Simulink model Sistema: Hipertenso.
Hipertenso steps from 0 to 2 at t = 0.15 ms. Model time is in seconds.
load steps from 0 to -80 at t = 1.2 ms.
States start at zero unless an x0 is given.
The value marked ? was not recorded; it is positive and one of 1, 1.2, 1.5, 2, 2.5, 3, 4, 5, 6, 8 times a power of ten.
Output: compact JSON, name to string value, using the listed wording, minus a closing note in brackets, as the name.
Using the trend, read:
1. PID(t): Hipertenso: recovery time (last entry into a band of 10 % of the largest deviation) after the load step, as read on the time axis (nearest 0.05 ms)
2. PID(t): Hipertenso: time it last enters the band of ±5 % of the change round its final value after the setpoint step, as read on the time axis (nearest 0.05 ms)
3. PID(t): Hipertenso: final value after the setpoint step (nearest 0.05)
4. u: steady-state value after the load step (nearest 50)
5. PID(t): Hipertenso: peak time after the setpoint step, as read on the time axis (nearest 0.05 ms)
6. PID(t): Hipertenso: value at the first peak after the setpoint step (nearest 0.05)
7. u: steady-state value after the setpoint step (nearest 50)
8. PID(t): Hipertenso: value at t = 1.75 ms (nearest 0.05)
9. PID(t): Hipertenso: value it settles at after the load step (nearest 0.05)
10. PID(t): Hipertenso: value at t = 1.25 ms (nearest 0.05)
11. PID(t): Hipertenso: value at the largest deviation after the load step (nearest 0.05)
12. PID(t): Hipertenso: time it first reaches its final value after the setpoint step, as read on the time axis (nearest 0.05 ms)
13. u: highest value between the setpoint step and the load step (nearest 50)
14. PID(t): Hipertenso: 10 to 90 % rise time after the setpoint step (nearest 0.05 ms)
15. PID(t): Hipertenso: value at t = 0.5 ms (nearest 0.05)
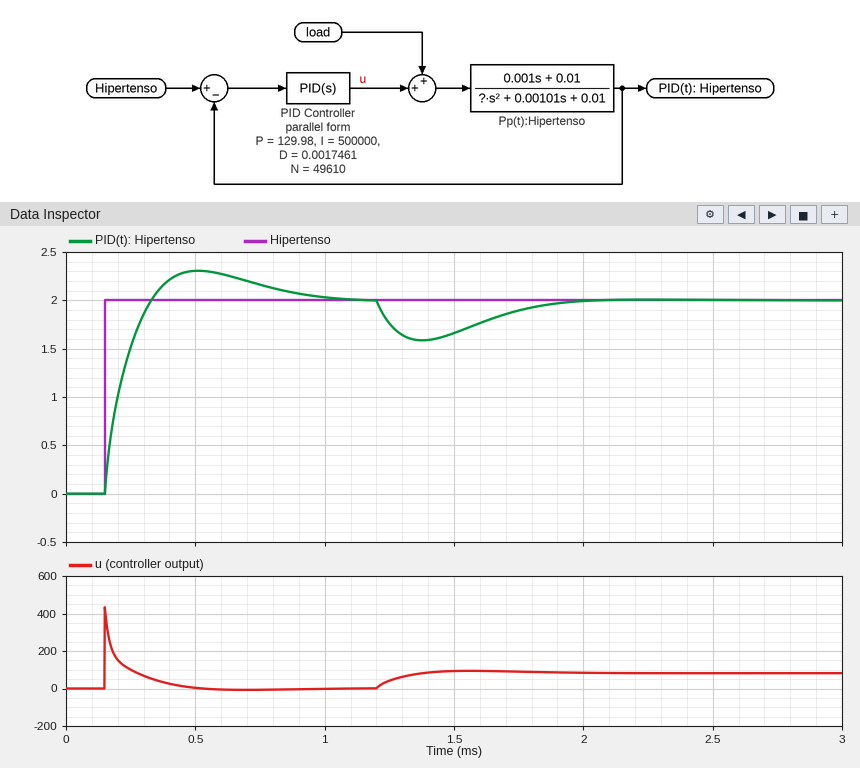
{"PID(t): Hipertenso: recovery time (last entry into a band of 10 % of the largest deviation) after the load step, as read on the time axis": "1.85 ms", "PID(t): Hipertenso: time it last enters the band of ±5 % of the change round its final value after the setpoint step, as read on the time axis": "0.85 ms", "PID(t): Hipertenso: final value after the setpoint step": "2.00", "u: steady-state value after the load step": "100", "PID(t): Hipertenso: peak time after the setpoint step, as read on the time axis": "0.50 ms", "PID(t): Hipertenso: value at the first peak after the setpoint step": "2.30", "u: steady-state value after the setpoint step": "0", "PID(t): Hipertenso: value at t = 1.75 ms": "1.90", "PID(t): Hipertenso: value it settles at after the load step": "2.00", "PID(t): Hipertenso: value at t = 1.25 ms": "1.75", "PID(t): Hipertenso: value at the largest deviation after the load step": "1.60", "PID(t): Hipertenso: time it first reaches its final value after the setpoint step, as read on the time axis": "0.35 ms", "u: highest value between the setpoint step and the load step": "450", "PID(t): Hipertenso: 10 to 90 % rise time after the setpoint step": "0.15 ms", "PID(t): Hipertenso: value at t = 0.5 ms": "2.30"}
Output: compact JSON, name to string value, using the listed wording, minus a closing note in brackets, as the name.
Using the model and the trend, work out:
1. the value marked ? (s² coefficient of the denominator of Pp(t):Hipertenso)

{"the value marked ? (s² coefficient of the denominator of Pp(t):Hipertenso)": "1.2e-05"}
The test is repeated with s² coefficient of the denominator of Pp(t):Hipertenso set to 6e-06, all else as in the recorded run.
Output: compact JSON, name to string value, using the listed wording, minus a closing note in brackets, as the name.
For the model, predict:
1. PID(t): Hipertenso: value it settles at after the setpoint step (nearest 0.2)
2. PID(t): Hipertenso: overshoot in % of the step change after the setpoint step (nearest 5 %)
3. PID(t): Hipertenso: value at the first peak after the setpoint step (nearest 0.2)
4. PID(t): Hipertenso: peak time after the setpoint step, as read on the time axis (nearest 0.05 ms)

{"PID(t): Hipertenso: value it settles at after the setpoint step": "2.0", "PID(t): Hipertenso: overshoot in % of the step change after the setpoint step": "10 %", "PID(t): Hipertenso: value at the first peak after the setpoint step": "2.2", "PID(t): Hipertenso: peak time after the setpoint step, as read on the time axis": "0.40 ms"}
